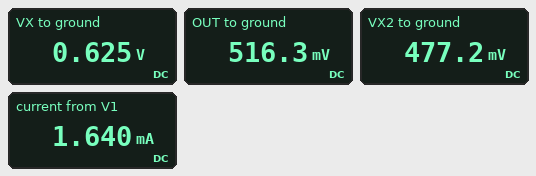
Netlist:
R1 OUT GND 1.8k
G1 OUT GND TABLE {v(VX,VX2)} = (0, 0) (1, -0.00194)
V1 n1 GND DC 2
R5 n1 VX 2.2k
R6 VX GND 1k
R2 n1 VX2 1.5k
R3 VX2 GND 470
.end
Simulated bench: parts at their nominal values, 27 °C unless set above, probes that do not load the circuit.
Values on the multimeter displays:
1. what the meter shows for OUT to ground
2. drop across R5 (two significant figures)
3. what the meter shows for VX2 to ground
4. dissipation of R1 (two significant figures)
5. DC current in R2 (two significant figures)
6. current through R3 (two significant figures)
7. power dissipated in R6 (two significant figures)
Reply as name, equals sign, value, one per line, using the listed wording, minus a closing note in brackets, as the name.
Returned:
what the meter shows for OUT to ground = 516.3 mV
drop across R5 = 1.4 V
what the meter shows for VX2 to ground = 477.2 mV
dissipation of R1 = 150 µW
DC current in R2 = 1.0 mA
current through R3 = 1.0 mA
power dissipated in R6 = 390 µW
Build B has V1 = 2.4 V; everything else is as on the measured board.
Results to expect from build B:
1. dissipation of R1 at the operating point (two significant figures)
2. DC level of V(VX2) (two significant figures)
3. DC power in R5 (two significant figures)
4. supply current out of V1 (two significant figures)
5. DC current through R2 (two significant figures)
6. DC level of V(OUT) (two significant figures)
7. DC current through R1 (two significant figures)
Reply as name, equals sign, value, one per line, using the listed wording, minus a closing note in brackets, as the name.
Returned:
dissipation of R1 at the operating point = 210 µW
DC level of V(VX2) = 570 mV
DC power in R5 = 1.2 mW
supply current out of V1 = 2.0 mA
DC current through R2 = 1.2 mA
DC level of V(OUT) = 620 mV
DC current through R1 = 340 µA
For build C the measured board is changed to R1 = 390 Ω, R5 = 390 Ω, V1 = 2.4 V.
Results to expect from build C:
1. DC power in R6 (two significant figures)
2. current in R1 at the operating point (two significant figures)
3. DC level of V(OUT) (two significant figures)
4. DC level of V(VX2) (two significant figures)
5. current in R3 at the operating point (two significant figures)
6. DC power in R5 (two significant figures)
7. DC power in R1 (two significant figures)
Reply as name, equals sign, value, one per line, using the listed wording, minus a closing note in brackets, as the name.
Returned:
DC power in R6 = 3.0 mW
current in R1 at the operating point = 1.9 mA
DC level of V(OUT) = 760 mV
DC level of V(VX2) = 570 mV
current in R3 at the operating point = 1.2 mA
DC power in R5 = 1.2 mW
DC power in R1 = 1.5 mW
